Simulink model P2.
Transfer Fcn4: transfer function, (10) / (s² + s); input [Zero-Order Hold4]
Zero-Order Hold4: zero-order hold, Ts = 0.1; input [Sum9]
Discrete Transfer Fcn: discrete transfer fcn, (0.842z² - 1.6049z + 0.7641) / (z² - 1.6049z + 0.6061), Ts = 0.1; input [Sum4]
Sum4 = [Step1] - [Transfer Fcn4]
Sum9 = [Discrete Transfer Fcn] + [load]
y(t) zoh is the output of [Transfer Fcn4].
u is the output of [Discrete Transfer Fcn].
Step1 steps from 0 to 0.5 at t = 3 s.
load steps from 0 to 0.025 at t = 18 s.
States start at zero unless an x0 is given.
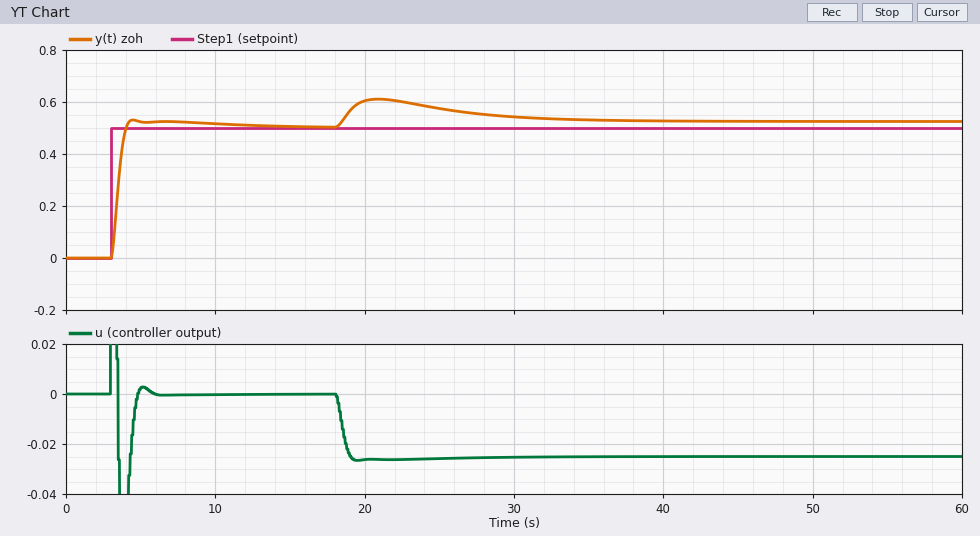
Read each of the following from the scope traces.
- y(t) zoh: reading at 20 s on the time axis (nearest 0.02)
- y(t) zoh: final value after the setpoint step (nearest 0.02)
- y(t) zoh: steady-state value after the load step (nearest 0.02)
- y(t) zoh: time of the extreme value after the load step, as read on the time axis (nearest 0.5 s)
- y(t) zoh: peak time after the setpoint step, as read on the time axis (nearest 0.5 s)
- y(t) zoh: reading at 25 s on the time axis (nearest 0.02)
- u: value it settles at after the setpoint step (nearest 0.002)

0.60
0.50
0.52
21.0 s
4.5 s
0.58
0.000
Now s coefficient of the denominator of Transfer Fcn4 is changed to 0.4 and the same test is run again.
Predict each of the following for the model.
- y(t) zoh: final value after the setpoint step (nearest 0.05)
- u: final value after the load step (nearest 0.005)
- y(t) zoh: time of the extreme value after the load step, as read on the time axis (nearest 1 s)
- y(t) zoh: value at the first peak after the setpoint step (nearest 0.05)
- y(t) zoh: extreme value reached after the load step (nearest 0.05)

0.50
-0.025
20 s
0.65
0.60
